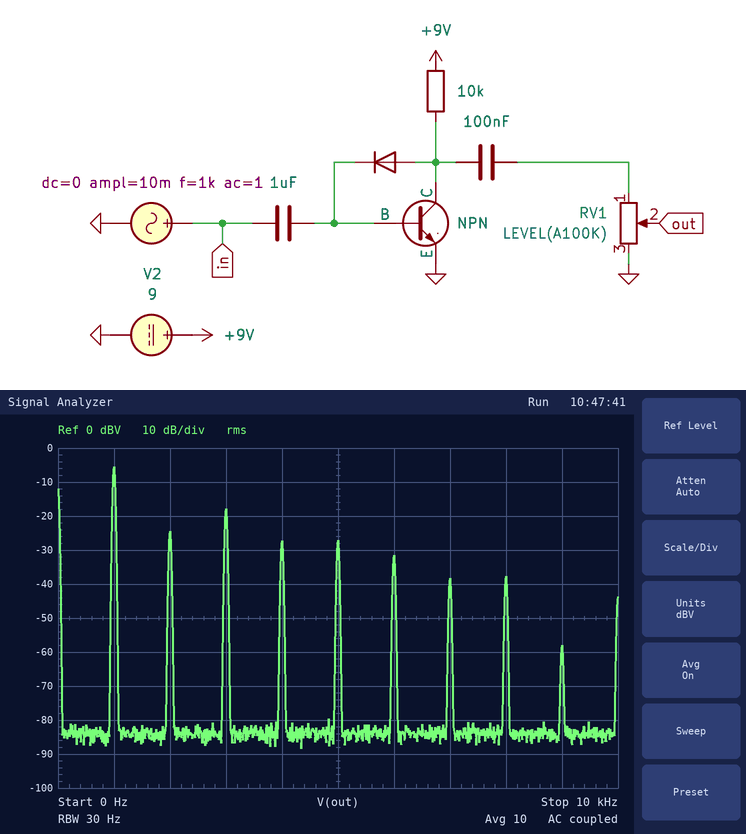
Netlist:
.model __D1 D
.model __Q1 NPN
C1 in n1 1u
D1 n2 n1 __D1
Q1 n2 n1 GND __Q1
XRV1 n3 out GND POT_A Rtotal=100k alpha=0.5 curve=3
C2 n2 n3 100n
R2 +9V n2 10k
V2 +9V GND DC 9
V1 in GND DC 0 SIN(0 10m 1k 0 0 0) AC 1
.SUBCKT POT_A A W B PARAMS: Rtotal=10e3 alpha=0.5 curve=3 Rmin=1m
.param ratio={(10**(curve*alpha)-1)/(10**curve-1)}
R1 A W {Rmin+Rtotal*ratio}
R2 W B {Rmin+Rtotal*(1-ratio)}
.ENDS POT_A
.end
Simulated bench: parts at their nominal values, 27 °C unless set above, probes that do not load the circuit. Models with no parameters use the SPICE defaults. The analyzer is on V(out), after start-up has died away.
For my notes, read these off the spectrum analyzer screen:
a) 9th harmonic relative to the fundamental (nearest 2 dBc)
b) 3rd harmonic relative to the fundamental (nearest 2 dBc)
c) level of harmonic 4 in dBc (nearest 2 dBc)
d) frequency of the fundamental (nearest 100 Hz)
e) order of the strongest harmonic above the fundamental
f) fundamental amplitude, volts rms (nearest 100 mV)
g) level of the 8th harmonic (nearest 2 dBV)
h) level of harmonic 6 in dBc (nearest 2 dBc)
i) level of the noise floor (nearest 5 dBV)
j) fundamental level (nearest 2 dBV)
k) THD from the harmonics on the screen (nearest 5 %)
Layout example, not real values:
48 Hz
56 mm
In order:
-52 dBc
-12 dBc
-22 dBc
1.0 kHz
3
500 mV
-38 dBV
-26 dBc
-85 dBV
-6 dBV
30 %
